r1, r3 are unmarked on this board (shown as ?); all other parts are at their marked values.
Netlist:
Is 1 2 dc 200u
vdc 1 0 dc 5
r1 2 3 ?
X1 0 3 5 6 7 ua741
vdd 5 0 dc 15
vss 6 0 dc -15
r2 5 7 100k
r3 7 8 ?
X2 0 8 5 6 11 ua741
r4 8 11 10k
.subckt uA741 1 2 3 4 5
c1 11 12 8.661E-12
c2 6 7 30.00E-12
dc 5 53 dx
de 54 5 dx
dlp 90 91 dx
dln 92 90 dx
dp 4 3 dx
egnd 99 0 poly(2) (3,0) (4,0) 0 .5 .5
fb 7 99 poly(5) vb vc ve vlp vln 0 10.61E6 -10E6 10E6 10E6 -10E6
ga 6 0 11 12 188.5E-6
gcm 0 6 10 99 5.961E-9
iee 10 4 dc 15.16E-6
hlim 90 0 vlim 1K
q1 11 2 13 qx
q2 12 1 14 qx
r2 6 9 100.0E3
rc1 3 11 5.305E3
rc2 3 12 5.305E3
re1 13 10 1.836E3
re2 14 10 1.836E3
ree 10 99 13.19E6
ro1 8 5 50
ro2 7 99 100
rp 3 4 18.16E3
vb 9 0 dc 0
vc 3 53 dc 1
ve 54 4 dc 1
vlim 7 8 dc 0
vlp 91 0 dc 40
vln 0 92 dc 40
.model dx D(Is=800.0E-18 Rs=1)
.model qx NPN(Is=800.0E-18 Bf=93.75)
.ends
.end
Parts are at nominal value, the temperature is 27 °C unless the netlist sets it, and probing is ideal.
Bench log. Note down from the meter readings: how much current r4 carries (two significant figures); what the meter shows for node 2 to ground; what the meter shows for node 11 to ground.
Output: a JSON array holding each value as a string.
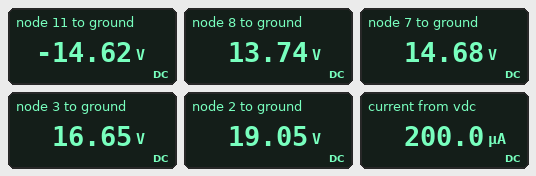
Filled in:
["2.8 mA", "19.05 V", "-14.62 V"]
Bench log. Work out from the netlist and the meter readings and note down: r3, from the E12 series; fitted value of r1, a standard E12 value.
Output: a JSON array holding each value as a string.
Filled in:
["330 Ω", "12 kΩ"]
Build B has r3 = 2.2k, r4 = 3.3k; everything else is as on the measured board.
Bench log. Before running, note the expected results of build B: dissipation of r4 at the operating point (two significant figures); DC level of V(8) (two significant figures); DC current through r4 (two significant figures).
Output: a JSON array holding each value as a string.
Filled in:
["94 mW", "3.0 V", "5.3 mA"]
